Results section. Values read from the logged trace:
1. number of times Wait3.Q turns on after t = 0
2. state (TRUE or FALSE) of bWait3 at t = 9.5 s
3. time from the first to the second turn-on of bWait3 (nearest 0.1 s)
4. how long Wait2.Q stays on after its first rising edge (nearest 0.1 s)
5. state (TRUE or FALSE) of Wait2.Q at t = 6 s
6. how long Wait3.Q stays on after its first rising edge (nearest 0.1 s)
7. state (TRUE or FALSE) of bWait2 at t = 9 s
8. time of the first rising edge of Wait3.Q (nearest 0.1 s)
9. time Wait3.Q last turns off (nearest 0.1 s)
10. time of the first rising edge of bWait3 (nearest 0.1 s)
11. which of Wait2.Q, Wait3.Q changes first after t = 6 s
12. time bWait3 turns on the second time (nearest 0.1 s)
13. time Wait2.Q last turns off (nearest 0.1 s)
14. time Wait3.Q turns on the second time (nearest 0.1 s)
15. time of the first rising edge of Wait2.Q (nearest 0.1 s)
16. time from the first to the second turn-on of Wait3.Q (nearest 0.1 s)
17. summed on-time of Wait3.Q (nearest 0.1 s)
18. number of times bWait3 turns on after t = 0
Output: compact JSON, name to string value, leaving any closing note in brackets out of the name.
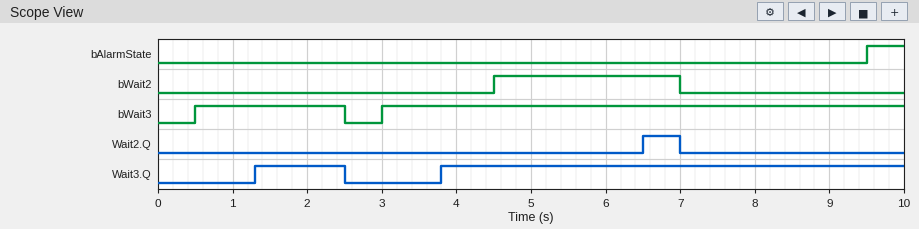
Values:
{"number of times Wait3.Q turns on after t = 0": "2", "state (TRUE or FALSE) of bWait3 at t = 9.5 s": "TRUE", "time from the first to the second turn-on of bWait3": "2.5 s", "how long Wait2.Q stays on after its first rising edge": "0.5 s", "state (TRUE or FALSE) of Wait2.Q at t = 6 s": "FALSE", "how long Wait3.Q stays on after its first rising edge": "1.2 s", "state (TRUE or FALSE) of bWait2 at t = 9 s": "FALSE", "time of the first rising edge of Wait3.Q": "1.3 s", "time Wait3.Q last turns off": "2.5 s", "time of the first rising edge of bWait3": "0.5 s", "which of Wait2.Q, Wait3.Q changes first after t = 6 s": "Wait2.Q", "time bWait3 turns on the second time": "3.0 s", "time Wait2.Q last turns off": "7.0 s", "time Wait3.Q turns on the second time": "3.8 s", "time of the first rising edge of Wait2.Q": "6.5 s", "time from the first to the second turn-on of Wait3.Q": "2.5 s", "summed on-time of Wait3.Q": "7.4 s", "number of times bWait3 turns on after t = 0": "2"}
